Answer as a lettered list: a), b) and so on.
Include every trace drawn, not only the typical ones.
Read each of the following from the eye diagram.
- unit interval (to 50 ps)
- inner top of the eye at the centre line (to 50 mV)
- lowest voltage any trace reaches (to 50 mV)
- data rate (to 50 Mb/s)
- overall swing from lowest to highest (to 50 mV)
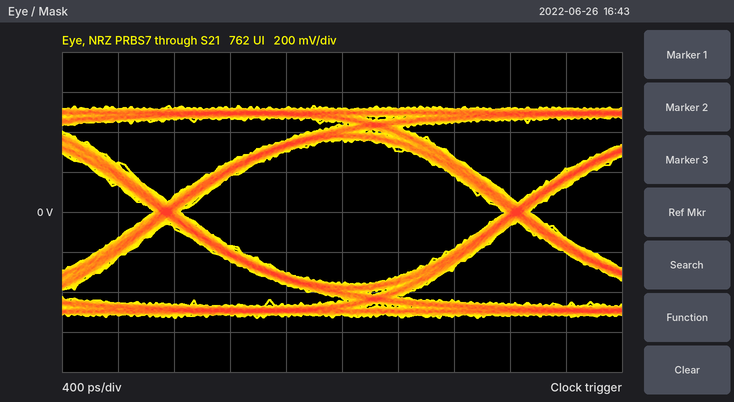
a) 2.50 ns
b) 350 mV
c) -550 mV
d) 400 Mb/s
e) 1.05 V
